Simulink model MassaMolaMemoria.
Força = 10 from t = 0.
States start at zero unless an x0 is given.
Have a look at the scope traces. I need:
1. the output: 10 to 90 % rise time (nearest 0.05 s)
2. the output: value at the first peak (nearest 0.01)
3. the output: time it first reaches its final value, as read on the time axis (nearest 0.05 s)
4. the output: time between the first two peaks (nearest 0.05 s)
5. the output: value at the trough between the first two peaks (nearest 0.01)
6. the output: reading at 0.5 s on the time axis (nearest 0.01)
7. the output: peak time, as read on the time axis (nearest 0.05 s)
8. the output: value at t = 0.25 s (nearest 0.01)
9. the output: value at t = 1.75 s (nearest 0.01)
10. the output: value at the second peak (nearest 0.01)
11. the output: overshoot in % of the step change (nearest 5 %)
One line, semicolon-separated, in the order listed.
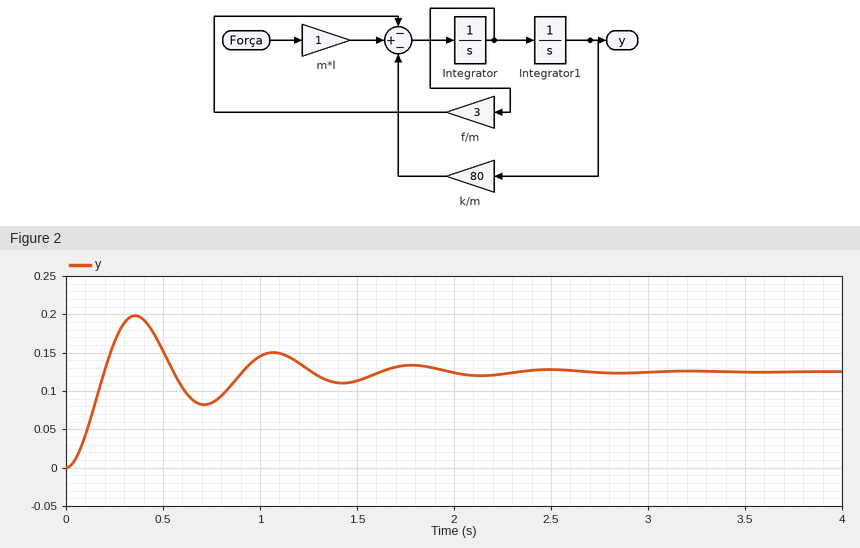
0.15 s; 0.20; 0.20 s; 0.70 s; 0.08; 0.15; 0.35 s; 0.16; 0.13; 0.15; 60 %
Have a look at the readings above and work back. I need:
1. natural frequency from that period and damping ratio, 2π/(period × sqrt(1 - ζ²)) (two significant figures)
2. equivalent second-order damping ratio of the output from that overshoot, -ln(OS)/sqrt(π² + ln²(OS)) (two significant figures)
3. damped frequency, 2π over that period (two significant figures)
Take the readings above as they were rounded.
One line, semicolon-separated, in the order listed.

9.1 rad/s; 0.16; 9.0 rad/s
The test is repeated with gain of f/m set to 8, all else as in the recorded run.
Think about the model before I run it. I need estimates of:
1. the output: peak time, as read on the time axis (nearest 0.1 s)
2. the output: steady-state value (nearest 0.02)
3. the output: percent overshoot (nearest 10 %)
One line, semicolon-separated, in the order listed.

0.4 s; 0.12; 20 %
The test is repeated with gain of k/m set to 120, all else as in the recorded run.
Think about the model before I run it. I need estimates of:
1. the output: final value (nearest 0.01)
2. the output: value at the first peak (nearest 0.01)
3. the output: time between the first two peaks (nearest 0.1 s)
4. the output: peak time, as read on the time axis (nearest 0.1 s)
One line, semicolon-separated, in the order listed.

0.08; 0.14; 0.6 s; 0.3 s
